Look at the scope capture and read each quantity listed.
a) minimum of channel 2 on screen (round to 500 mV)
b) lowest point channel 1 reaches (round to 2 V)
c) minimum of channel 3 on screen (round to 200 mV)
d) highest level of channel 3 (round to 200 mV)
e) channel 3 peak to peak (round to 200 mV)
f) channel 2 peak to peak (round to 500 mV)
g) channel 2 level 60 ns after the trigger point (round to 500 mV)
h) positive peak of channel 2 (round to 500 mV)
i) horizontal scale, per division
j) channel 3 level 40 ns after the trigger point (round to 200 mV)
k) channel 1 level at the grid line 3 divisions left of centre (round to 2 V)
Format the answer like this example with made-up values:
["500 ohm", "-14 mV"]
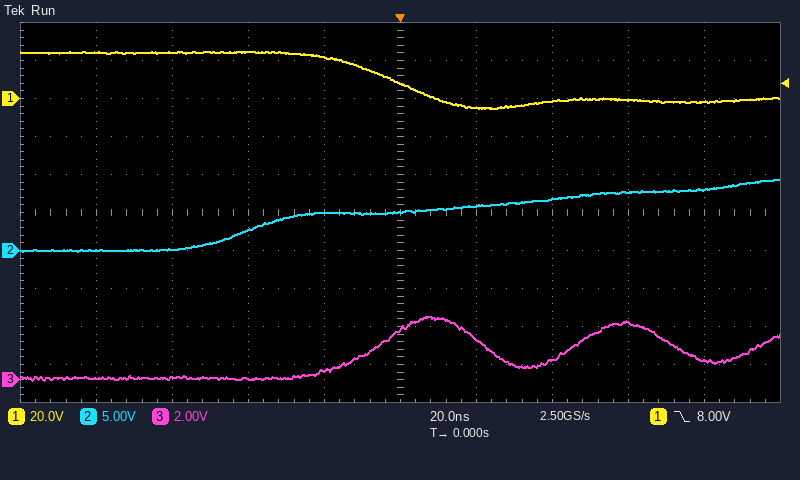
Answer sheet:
["0.0 V", "-6 V", "0.0 V", "3.4 V", "3.4 V", "9.5 V", "7.5 V", "9.5 V", "20 ns", "1.0 V", "24 V"]
